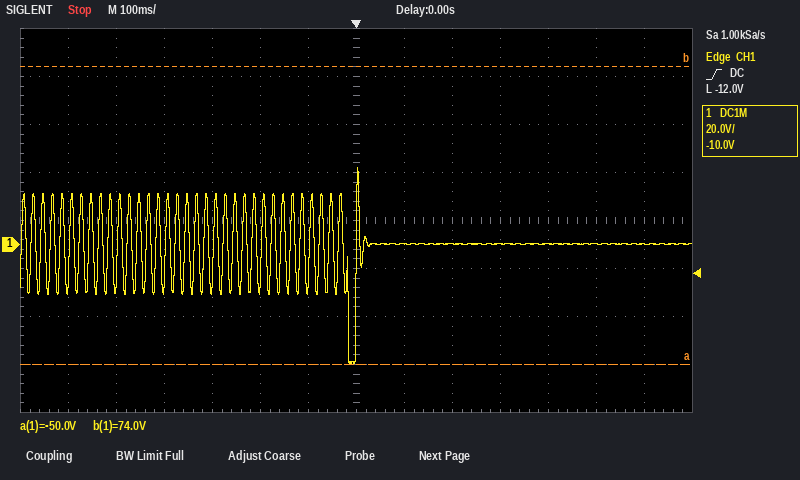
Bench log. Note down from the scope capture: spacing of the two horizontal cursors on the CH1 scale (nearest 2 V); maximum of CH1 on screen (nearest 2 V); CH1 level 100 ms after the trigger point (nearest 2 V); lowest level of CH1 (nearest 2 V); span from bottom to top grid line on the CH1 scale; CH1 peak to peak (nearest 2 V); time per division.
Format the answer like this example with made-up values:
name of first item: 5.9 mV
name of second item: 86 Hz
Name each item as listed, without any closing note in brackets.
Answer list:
spacing of the two horizontal cursors on the CH1 scale: 124 V
maximum of CH1 on screen: 32 V
CH1 level 100 ms after the trigger point: 0 V
lowest level of CH1: -50 V
span from bottom to top grid line on the CH1 scale: 160 V
CH1 peak to peak: 82 V
time per division: 100 ms
